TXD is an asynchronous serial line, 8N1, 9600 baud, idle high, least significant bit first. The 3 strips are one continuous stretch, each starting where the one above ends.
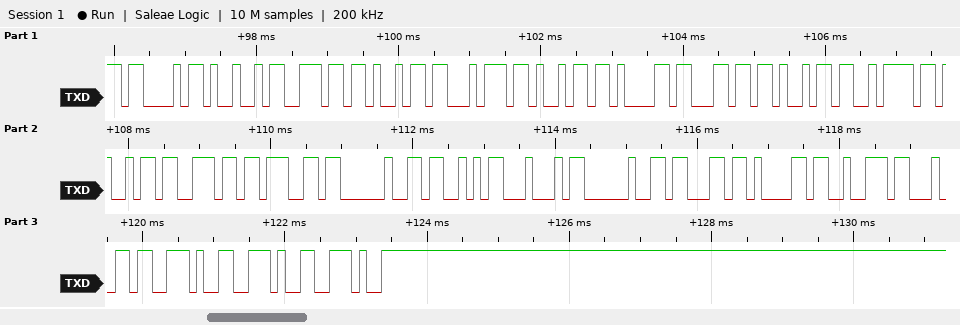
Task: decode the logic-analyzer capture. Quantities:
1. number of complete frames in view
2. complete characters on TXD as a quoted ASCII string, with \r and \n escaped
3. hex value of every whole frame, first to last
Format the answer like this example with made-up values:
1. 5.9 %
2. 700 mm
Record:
1. 24
2. "CInitializing SD card..."
3. 0x43 0x49 0x6E 0x69 0x74 0x69 0x61 0x6C 0x69 0x7A 0x69 0x6E 0x67 0x20 0x53 0x44 0x20 0x63 0x61 0x72 0x64 0x2E 0x2E 0x2E
